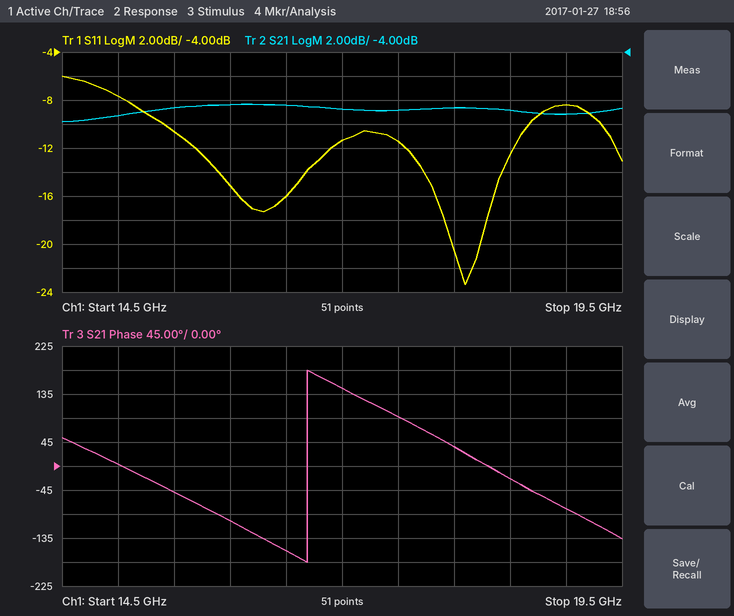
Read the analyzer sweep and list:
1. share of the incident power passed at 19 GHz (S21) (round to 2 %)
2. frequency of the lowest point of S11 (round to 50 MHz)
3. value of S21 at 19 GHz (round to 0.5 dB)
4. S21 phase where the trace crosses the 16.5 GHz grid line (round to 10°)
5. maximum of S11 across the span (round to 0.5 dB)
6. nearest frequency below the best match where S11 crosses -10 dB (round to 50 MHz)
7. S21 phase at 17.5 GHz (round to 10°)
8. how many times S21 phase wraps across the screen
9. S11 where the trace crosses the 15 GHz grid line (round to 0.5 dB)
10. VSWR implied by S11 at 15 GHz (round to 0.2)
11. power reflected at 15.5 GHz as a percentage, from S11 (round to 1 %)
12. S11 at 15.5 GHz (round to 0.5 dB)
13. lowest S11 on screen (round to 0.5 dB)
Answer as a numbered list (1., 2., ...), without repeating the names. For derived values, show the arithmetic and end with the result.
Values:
1. 10^(-9/10) ≈ 12.6 %, so 12 % to the nearest 2 %
2. 18.10 GHz
3. -9.0 dB
4. -160°
5. -6.0 dB
6. 15.40 GHz
7. 90°
8. 1
9. -7.5 dB
10. |Γ| = 10^(-7.5/20) = 0.4217; VSWR = (1 + 0.4217)/(1 − 0.4217) ≈ 2.46, so 2.4 to the nearest 0.2
11. 10^(-10.5/10) ≈ 9 %
12. -10.5 dB
13. -23.5 dB
